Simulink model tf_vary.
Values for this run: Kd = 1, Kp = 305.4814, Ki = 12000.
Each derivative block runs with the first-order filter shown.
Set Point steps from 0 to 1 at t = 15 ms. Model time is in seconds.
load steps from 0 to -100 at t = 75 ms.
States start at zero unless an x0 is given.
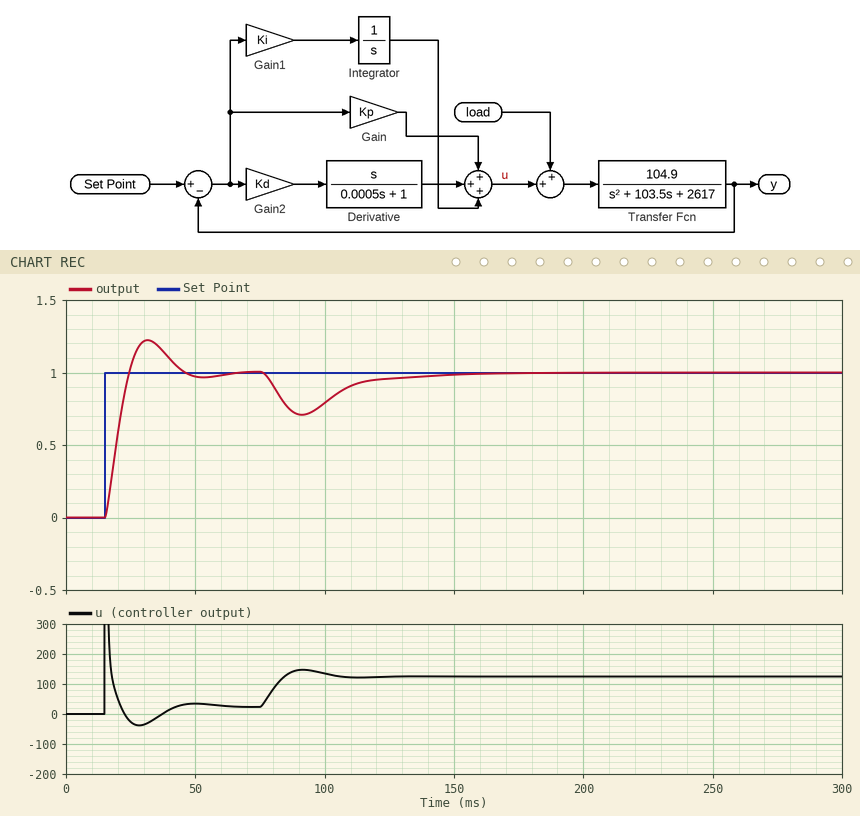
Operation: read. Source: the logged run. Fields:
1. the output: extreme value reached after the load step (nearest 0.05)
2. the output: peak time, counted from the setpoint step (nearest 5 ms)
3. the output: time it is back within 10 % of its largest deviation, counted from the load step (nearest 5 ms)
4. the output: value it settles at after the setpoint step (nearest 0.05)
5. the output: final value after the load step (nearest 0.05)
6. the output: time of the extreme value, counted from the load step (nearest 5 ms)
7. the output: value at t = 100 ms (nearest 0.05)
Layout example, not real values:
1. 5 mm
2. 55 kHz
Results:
1. 0.70
2. 15 ms
3. 60 ms
4. 1.00
5. 1.00
6. 15 ms
7. 0.80
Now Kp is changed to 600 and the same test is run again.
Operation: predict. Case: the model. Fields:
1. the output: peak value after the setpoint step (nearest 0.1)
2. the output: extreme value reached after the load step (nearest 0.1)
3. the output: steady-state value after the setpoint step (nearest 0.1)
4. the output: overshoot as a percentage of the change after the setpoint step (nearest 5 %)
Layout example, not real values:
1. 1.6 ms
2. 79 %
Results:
1. 1.3
2. 0.8
3. 1.0
4. 30 %
